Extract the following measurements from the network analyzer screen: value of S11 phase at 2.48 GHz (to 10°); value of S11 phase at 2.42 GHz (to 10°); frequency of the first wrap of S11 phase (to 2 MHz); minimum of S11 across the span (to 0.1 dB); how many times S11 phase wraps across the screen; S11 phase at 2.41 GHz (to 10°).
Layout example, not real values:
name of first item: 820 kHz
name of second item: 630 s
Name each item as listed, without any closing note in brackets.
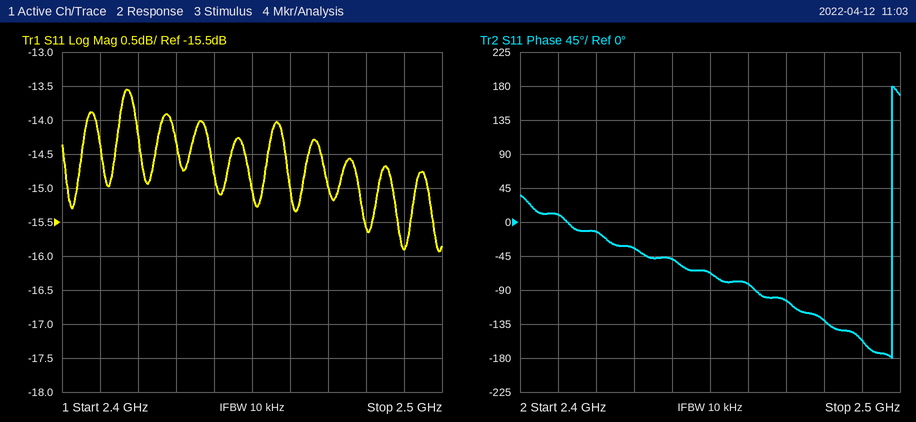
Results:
value of S11 phase at 2.48 GHz: -130°
value of S11 phase at 2.42 GHz: -10°
frequency of the first wrap of S11 phase: 2.498 GHz
minimum of S11 across the span: -15.9 dB
how many times S11 phase wraps across the screen: 1
S11 phase at 2.41 GHz: 10°
